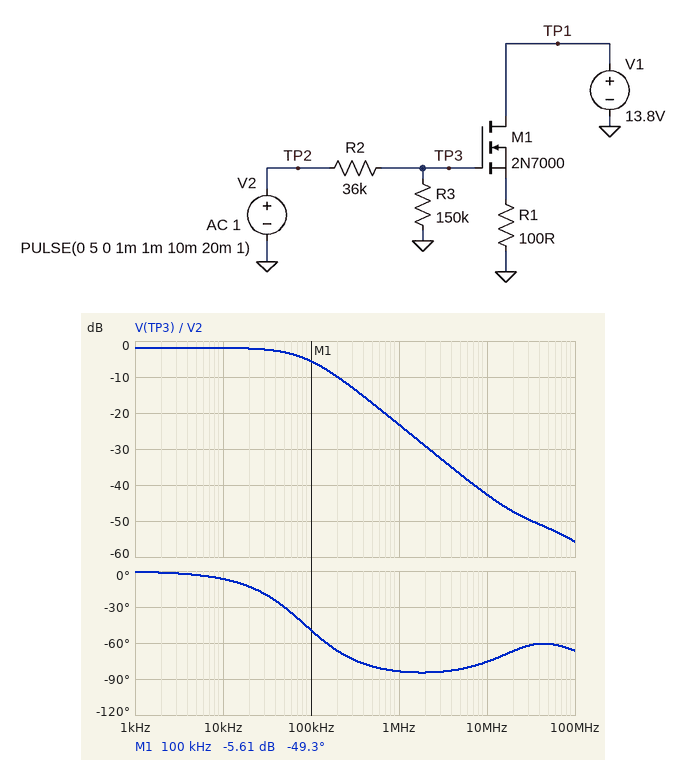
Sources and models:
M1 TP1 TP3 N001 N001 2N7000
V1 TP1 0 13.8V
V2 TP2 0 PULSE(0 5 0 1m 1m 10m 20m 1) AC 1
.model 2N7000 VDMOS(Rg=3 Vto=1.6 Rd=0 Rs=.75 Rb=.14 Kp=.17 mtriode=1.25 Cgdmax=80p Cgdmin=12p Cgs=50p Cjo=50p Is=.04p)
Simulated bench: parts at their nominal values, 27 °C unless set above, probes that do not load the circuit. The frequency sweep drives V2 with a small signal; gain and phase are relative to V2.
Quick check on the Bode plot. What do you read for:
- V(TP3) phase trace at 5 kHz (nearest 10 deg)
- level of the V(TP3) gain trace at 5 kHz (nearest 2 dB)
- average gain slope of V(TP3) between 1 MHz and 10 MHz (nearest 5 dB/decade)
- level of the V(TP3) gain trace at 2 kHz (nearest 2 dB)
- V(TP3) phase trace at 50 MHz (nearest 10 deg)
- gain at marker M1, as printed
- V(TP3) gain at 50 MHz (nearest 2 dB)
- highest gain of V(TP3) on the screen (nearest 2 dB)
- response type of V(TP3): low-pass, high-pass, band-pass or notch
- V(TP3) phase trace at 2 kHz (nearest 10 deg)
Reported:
0 deg
-2 dB
-20 dB/decade
-2 dB
-60 deg
-5.61 dB
-52 dB
-2 dB
low-pass
0 deg
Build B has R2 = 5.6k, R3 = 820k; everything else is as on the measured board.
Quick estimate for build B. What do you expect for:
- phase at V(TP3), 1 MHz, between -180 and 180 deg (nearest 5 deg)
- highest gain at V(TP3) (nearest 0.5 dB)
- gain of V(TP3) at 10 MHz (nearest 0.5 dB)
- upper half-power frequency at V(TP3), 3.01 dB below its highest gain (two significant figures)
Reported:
-65 deg
0 dB
-26.5 dB
440 kHz
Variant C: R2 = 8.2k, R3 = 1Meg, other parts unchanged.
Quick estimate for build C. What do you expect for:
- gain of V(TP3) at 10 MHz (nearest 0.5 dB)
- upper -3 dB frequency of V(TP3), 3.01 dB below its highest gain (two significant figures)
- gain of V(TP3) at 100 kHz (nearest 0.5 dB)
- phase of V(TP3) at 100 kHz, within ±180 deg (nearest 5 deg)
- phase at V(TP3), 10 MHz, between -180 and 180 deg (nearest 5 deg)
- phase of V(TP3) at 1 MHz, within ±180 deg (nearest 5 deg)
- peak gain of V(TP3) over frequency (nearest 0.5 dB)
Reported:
-30.0 dB
300 kHz
-0.5 dB
-20 deg
-75 deg
-70 deg
0 dB
